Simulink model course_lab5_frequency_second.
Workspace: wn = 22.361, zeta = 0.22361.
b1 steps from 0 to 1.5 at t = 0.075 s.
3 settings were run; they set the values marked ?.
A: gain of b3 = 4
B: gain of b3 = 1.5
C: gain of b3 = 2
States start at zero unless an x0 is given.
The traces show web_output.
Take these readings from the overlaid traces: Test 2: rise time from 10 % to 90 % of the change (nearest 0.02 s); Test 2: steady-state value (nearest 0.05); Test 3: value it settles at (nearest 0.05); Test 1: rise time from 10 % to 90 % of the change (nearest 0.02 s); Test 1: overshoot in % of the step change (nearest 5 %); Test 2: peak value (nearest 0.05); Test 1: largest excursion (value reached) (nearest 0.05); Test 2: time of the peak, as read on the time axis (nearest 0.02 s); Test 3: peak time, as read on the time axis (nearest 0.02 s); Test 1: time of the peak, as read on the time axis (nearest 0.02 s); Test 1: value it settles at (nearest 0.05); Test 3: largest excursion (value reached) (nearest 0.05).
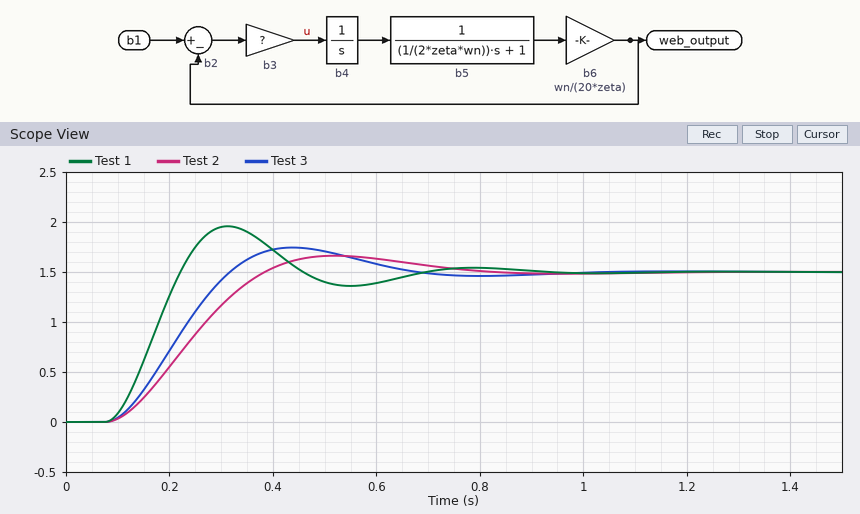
0.20 s
1.50
1.50
0.10 s
30 %
1.65
1.95
0.52 s
0.44 s
0.32 s
1.50
1.75
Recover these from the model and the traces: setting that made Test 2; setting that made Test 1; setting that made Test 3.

B
A
C
